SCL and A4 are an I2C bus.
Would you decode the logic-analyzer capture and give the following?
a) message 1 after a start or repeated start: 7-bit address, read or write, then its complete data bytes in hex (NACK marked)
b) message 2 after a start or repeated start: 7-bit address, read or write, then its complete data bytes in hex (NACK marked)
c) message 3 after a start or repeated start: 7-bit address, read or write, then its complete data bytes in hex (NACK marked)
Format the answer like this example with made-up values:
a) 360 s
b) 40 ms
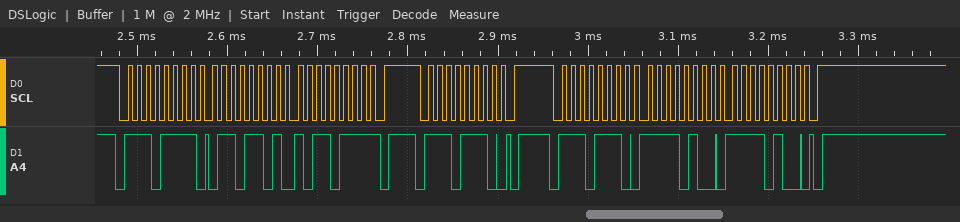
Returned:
a) 0x77 read: 6D B7 NACK
b) 0x77 write
c) 0x77 write: F4 F4
